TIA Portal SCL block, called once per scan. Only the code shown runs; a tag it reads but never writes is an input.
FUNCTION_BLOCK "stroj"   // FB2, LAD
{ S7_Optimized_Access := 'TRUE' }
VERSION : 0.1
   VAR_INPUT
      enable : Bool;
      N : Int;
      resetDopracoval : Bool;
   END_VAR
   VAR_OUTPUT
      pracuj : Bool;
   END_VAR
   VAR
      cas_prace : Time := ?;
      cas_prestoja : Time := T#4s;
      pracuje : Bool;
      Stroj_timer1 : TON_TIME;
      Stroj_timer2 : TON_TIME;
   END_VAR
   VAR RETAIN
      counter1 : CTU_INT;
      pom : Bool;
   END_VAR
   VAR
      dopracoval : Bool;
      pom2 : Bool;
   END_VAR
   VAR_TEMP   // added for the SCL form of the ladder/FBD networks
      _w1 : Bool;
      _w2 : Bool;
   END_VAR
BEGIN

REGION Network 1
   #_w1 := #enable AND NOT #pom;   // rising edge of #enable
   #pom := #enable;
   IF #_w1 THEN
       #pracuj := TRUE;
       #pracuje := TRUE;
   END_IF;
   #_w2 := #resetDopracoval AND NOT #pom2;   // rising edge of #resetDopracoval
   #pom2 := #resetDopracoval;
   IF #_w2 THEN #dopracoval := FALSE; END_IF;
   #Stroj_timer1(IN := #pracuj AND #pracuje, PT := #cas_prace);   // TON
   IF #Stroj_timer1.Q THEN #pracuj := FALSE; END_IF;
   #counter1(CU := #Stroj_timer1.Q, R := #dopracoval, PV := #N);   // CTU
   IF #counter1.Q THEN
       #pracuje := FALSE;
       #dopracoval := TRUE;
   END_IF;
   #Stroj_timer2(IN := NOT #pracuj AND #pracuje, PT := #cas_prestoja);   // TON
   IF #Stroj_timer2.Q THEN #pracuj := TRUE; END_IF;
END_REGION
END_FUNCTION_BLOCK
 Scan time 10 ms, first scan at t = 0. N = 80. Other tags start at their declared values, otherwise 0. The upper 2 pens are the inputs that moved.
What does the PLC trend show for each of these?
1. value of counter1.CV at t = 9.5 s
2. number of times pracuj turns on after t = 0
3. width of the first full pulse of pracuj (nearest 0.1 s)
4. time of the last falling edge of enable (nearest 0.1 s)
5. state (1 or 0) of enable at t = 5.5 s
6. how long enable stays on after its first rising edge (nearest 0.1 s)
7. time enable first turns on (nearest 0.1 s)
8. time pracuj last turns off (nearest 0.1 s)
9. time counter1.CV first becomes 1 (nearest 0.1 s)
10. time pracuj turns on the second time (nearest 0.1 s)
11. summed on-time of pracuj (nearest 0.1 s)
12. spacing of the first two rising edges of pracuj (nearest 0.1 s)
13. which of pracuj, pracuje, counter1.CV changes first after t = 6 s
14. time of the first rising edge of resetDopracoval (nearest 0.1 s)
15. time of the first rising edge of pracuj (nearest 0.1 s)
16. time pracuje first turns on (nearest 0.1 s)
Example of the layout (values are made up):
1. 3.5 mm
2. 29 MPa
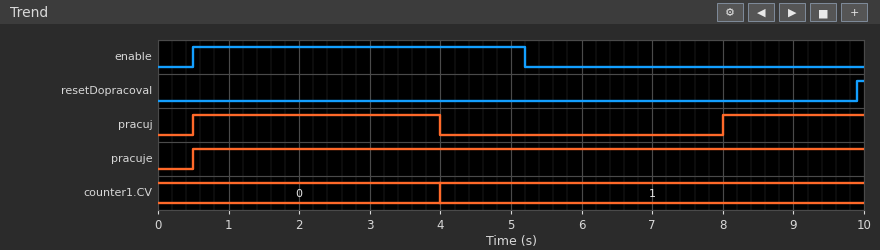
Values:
1. 1
2. 2
3. 3.5 s
4. 5.2 s
5. 0
6. 4.7 s
7. 0.5 s
8. 4.0 s
9. 4.0 s
10. 8.0 s
11. 5.5 s
12. 7.5 s
13. pracuj
14. 9.9 s
15. 0.5 s
16. 0.5 s
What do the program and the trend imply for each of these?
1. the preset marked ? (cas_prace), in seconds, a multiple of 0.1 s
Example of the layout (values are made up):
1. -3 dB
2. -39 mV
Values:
1. 3.5 s
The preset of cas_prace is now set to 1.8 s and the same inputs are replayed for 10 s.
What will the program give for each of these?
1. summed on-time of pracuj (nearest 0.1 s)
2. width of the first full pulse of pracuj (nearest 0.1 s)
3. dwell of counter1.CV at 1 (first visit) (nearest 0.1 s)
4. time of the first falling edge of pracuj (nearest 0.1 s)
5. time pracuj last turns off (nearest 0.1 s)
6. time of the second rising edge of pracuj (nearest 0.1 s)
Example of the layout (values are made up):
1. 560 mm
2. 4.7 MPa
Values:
1. 3.6 s
2. 1.8 s
3. 5.8 s
4. 2.3 s
5. 8.1 s
6. 6.3 s
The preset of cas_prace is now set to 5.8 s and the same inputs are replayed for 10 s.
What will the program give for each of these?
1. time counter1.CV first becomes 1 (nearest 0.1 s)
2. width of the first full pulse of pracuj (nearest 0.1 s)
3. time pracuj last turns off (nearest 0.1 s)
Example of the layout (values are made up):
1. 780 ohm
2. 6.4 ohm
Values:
1. 6.3 s
2. 5.8 s
3. 6.3 s
